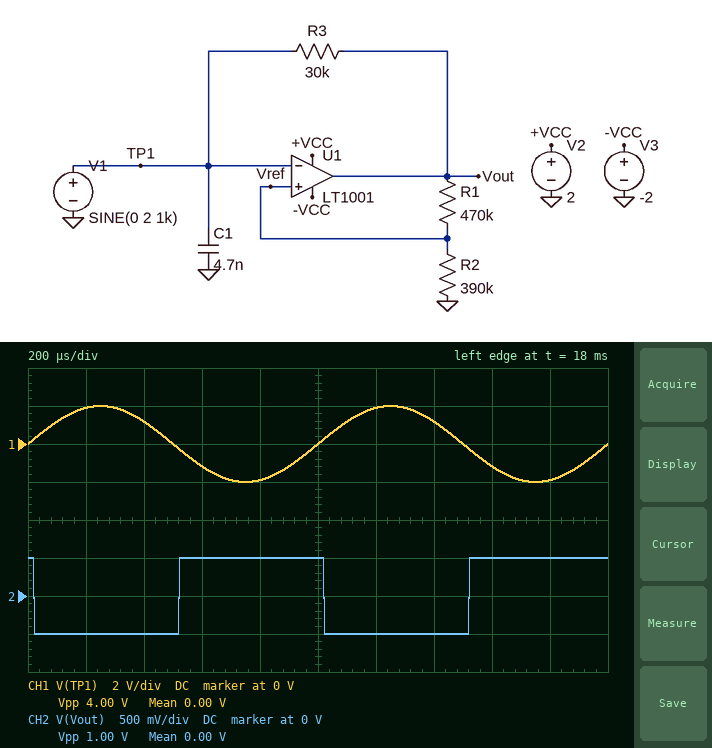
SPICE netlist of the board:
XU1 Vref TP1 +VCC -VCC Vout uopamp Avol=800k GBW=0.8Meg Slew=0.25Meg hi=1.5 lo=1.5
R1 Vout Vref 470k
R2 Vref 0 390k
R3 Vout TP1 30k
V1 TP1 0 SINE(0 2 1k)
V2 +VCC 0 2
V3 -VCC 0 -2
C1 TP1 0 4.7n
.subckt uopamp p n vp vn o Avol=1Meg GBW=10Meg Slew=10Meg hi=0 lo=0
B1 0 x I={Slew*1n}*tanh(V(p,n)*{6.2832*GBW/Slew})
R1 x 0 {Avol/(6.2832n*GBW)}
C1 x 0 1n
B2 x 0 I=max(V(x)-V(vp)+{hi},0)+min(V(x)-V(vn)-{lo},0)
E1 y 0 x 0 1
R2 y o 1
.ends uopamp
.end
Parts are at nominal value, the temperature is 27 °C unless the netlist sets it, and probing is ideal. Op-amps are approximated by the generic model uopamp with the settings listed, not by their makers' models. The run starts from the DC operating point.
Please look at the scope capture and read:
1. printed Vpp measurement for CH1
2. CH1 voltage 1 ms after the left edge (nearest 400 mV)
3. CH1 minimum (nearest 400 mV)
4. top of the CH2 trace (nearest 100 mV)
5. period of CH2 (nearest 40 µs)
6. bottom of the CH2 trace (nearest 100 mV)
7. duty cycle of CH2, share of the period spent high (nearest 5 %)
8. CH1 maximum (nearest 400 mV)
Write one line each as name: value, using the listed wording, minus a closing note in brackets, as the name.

printed Vpp measurement for CH1: 4.00 V
CH1 voltage 1 ms after the left edge: 0 V
CH1 minimum: -2.0 V
top of the CH2 trace: 500 mV
period of CH2: 1.00 ms
bottom of the CH2 trace: -500 mV
duty cycle of CH2, share of the period spent high: 50 %
CH1 maximum: 2.0 V
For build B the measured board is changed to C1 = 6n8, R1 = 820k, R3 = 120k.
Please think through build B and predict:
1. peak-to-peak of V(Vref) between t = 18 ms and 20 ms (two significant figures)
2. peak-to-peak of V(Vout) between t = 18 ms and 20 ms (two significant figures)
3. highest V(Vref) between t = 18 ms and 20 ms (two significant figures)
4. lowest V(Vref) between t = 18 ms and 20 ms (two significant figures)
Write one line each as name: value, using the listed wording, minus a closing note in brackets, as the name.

peak-to-peak of V(Vref) between t = 18 ms and 20 ms: 320 mV
peak-to-peak of V(Vout) between t = 18 ms and 20 ms: 1.0 V
highest V(Vref) between t = 18 ms and 20 ms: 160 mV
lowest V(Vref) between t = 18 ms and 20 ms: -160 mV
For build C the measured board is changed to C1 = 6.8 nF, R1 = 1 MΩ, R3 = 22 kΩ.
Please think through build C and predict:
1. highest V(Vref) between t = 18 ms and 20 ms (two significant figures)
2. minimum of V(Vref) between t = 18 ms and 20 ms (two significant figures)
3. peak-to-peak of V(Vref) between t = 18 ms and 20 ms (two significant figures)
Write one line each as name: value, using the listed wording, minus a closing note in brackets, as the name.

highest V(Vref) between t = 18 ms and 20 ms: 140 mV
minimum of V(Vref) between t = 18 ms and 20 ms: -140 mV
peak-to-peak of V(Vref) between t = 18 ms and 20 ms: 280 mV
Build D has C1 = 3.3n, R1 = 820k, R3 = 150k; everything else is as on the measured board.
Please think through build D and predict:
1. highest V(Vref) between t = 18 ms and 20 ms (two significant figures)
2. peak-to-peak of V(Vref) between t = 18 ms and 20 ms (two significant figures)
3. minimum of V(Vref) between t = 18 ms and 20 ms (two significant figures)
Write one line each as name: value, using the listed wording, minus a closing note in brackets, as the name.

highest V(Vref) between t = 18 ms and 20 ms: 160 mV
peak-to-peak of V(Vref) between t = 18 ms and 20 ms: 320 mV
minimum of V(Vref) between t = 18 ms and 20 ms: -160 mV
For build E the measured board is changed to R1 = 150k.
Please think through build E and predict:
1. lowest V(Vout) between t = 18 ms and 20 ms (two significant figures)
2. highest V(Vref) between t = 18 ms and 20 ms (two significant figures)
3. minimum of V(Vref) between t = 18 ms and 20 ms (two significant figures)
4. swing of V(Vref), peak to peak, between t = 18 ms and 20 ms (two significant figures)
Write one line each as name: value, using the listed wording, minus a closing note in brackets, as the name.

lowest V(Vout) between t = 18 ms and 20 ms: -500 mV
highest V(Vref) between t = 18 ms and 20 ms: 360 mV
minimum of V(Vref) between t = 18 ms and 20 ms: -360 mV
swing of V(Vref), peak to peak, between t = 18 ms and 20 ms: 720 mV
